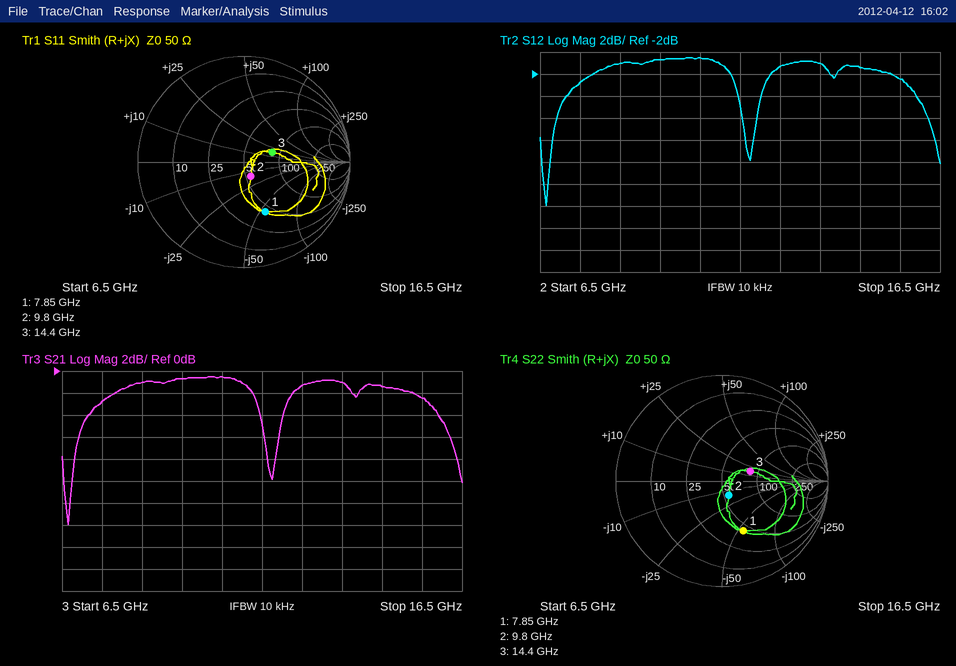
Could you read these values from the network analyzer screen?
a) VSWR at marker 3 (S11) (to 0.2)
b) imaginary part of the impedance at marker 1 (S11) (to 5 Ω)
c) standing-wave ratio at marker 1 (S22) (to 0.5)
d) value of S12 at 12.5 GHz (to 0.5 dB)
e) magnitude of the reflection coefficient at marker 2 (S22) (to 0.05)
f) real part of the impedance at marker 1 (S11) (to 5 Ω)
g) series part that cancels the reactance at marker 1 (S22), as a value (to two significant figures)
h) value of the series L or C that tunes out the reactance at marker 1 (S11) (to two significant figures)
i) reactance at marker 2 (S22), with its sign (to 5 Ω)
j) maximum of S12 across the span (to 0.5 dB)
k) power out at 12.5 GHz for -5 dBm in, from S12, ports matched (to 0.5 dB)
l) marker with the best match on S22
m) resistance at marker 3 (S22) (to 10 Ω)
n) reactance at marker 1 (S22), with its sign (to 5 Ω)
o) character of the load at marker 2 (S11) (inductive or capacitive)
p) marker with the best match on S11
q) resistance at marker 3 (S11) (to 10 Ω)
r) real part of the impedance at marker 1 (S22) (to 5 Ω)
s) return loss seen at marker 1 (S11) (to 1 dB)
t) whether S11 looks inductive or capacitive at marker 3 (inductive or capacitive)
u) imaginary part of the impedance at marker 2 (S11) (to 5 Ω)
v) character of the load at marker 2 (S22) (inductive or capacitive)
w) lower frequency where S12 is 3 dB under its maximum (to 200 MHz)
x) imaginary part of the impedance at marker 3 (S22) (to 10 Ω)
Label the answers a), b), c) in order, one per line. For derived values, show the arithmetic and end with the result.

a) 1.8
b) -55 Ω
c) 3.0
d) -1.5 dB
e) 0.15
f) 45 Ω
g) L = 55 Ω/(2π × 7.85 GHz) ≈ 1.1 nH
h) L = 55 Ω/(2π × 7.85 GHz) ≈ 1.1 nH
i) -15 Ω
j) -0.5 dB
k) -5 dBm + (-1.5 dB) = -6.5 dBm
l) marker 2
m) 80 Ω
n) -55 Ω
o) capacitive
p) marker 2
q) 80 Ω
r) 45 Ω
s) 6 dB
t) inductive
u) -15 Ω
v) capacitive
w) 7.2 GHz
x) +20 Ω
